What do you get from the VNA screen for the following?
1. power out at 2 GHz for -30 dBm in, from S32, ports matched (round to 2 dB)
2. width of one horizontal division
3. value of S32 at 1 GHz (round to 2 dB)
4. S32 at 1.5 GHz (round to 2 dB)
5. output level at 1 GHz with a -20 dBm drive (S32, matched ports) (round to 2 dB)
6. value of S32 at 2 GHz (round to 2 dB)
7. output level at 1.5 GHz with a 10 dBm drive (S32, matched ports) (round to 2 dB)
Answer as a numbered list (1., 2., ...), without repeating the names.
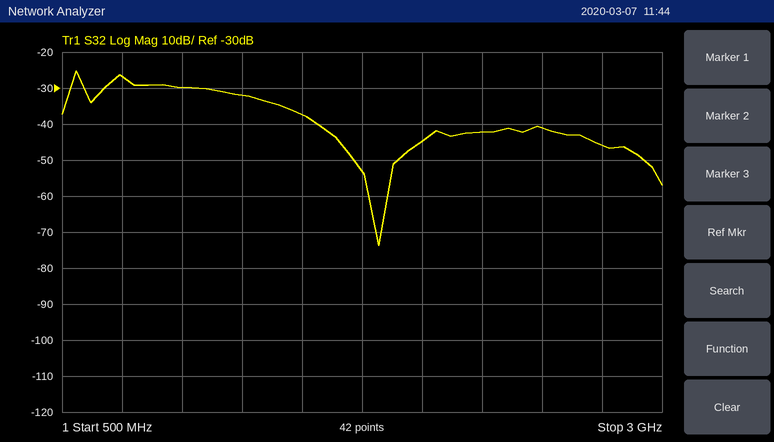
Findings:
1. -74 dBm
2. 250 MHz
3. -30 dB
4. -38 dB
5. -50 dBm
6. -44 dB
7. -28 dBm
